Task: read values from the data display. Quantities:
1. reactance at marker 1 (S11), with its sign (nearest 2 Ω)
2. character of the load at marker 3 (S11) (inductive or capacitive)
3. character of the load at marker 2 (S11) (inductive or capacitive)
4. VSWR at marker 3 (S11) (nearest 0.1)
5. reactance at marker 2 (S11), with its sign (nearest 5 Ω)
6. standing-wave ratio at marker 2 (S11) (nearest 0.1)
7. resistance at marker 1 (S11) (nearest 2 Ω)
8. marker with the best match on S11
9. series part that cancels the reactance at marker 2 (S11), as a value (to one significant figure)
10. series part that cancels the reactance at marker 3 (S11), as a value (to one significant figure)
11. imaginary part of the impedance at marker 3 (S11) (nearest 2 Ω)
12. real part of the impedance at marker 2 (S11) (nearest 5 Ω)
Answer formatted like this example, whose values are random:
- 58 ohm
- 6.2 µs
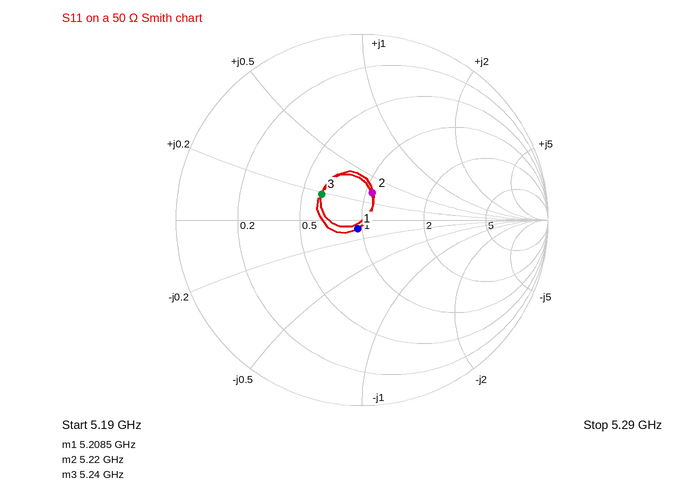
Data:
- -4 Ω
- inductive
- inductive
- 1.7
- +15 Ω
- 1.4
- 48 Ω
- marker 1
- 2 pF
- 3 pF
- +10 Ω
- 55 Ω
